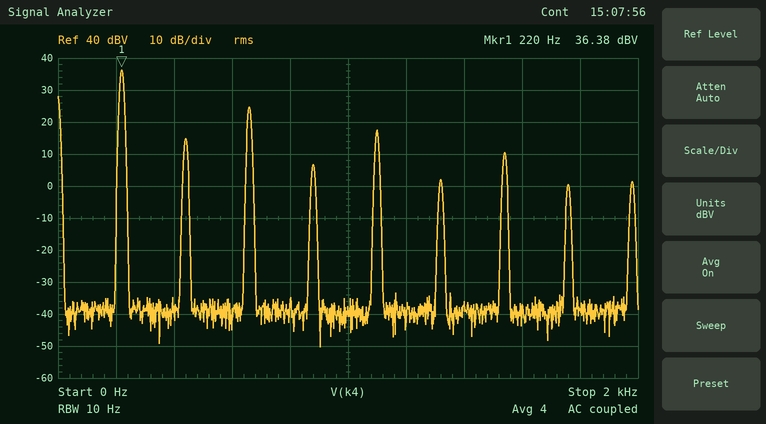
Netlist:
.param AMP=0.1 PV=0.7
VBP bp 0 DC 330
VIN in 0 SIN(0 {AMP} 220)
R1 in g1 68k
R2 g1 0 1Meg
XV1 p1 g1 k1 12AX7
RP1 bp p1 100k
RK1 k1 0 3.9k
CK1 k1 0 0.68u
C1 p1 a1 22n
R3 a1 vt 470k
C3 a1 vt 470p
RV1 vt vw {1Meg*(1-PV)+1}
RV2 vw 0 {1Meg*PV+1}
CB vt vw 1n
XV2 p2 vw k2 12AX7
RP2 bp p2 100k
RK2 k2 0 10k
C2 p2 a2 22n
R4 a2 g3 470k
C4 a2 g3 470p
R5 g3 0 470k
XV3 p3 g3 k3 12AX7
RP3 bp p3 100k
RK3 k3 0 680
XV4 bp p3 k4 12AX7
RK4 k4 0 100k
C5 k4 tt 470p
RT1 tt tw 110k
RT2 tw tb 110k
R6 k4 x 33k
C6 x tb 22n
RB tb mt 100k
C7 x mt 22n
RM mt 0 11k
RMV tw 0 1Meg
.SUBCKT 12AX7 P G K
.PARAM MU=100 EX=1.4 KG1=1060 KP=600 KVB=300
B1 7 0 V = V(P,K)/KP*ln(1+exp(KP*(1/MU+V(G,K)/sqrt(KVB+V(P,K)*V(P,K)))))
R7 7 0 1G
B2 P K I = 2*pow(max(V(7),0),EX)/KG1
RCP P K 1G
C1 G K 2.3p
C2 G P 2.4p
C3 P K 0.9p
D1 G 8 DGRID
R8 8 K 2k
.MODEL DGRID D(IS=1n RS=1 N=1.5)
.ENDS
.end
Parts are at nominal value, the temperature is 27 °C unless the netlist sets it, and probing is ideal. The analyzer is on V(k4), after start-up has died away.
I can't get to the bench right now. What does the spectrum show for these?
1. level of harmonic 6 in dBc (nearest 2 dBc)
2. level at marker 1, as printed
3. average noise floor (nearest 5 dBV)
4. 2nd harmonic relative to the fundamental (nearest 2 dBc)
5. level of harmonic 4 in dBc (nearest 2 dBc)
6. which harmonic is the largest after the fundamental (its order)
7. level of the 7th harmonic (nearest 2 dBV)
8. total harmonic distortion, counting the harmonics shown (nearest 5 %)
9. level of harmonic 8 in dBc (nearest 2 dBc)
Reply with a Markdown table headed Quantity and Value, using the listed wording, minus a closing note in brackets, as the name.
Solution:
| Quantity | Value |
|---|---|
| level of harmonic 6 in dBc | -34 dBc |
| level at marker 1, as printed | 36.38 dBV |
| average noise floor | -40 dBV |
| 2nd harmonic relative to the fundamental | -22 dBc |
| level of harmonic 4 in dBc | -30 dBc |
| which harmonic is the largest after the fundamental | 3 |
| level of the 7th harmonic | 10 dBV |
| total harmonic distortion, counting the harmonics shown | 30 % |
| level of harmonic 8 in dBc | -36 dBc |
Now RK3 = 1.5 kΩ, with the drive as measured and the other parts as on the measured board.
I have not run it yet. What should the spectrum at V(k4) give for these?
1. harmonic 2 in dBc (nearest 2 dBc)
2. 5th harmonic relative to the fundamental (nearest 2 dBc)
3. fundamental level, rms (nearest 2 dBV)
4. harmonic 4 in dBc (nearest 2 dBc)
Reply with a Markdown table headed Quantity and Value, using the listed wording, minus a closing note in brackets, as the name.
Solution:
| Quantity | Value |
|---|---|
| harmonic 2 in dBc | -18 dBc |
| 5th harmonic relative to the fundamental | -24 dBc |
| fundamental level, rms | 36 dBV |
| harmonic 4 in dBc | -22 dBc |
